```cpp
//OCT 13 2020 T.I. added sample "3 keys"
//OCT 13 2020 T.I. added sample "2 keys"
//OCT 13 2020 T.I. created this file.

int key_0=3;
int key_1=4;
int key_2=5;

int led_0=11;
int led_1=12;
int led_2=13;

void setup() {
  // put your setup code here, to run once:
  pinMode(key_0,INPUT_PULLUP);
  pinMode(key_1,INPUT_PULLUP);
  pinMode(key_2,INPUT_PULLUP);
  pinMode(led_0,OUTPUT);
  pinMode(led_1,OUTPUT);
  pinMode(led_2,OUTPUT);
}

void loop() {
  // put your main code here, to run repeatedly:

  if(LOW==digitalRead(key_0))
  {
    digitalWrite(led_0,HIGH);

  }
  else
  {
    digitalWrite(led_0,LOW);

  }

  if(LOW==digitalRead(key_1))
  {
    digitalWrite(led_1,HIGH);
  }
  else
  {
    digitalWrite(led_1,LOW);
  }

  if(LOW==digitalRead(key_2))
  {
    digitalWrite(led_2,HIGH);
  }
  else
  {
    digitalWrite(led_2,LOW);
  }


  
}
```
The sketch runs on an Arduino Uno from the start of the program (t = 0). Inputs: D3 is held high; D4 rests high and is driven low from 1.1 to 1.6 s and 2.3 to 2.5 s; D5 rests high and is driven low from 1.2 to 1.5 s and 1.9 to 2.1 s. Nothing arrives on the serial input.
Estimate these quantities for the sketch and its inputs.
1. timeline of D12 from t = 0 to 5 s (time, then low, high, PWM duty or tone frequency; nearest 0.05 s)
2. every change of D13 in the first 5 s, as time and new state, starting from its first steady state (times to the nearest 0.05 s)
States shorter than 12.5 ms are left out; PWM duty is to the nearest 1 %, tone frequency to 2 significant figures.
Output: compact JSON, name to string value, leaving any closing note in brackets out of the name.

{"timeline of D12 from t = 0 to 5 s": "0 s low; 1.1 s high; 1.6 s low; 2.3 s high; 2.5 s low", "every change of D13 in the first 5 s, as time and new state, starting from its first steady state": "0 s low; 1.2 s high; 1.5 s low; 1.9 s high; 2.1 s low"}
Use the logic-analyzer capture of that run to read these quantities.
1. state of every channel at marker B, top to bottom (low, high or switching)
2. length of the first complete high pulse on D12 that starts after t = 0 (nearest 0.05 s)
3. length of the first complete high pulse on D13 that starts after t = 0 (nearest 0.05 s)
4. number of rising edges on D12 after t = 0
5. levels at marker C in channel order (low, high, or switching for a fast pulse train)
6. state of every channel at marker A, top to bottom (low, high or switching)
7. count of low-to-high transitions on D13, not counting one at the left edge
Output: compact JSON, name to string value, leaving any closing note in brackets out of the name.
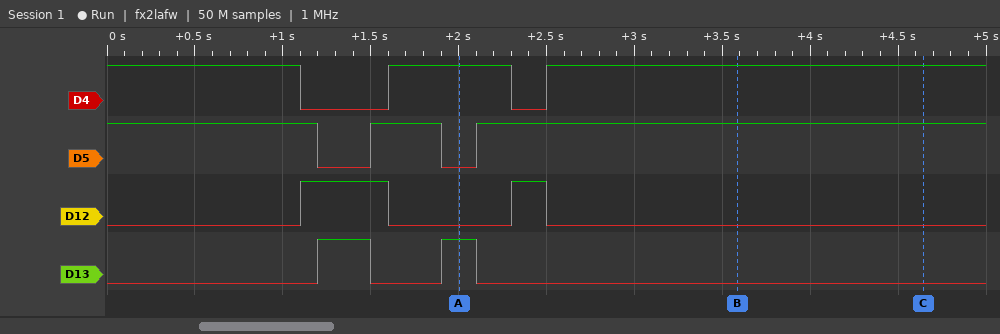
{"state of every channel at marker B, top to bottom": "D4 high, D5 high, D12 low, D13 low", "length of the first complete high pulse on D12 that starts after t = 0": "0.50 s", "length of the first complete high pulse on D13 that starts after t = 0": "0.30 s", "number of rising edges on D12 after t = 0": "2", "levels at marker C in channel order": "D4 high, D5 high, D12 low, D13 low", "state of every channel at marker A, top to bottom": "D4 high, D5 low, D12 low, D13 high", "count of low-to-high transitions on D13, not counting one at the left edge": "2"}
